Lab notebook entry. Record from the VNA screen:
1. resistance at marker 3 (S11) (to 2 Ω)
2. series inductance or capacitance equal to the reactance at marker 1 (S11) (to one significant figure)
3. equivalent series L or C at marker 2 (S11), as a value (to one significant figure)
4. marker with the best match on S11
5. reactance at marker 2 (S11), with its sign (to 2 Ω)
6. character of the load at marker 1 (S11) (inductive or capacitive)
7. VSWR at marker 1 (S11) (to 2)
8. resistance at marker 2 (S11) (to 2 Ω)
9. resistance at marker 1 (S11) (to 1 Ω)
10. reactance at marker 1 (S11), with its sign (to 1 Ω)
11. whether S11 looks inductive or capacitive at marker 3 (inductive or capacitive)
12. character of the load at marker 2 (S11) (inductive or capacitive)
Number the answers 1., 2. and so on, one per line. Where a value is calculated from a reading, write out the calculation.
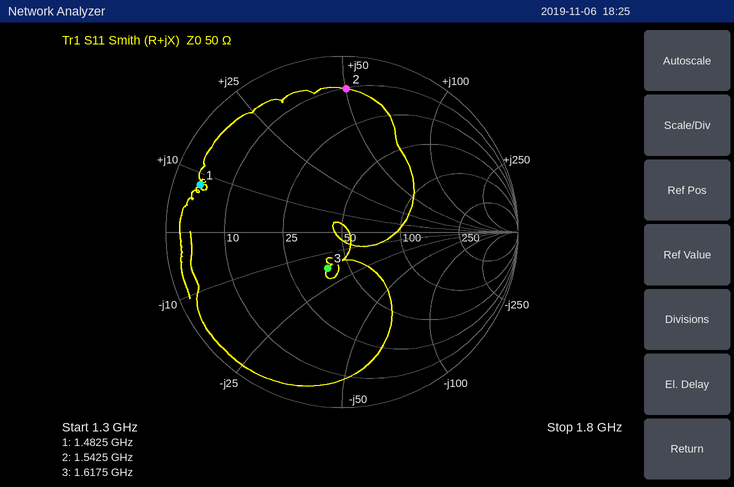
1. 40 Ω
2. L = 8 Ω/(2π × 1.4825 GHz) ≈ 859 pH, so 900 pH to one significant figure
3. L = 50 Ω/(2π × 1.5425 GHz) ≈ 5 nH
4. marker 3
5. +50 Ω
6. inductive
7. 12
8. 10 Ω
9. 4 Ω
10. +8 Ω
11. capacitive
12. inductive
